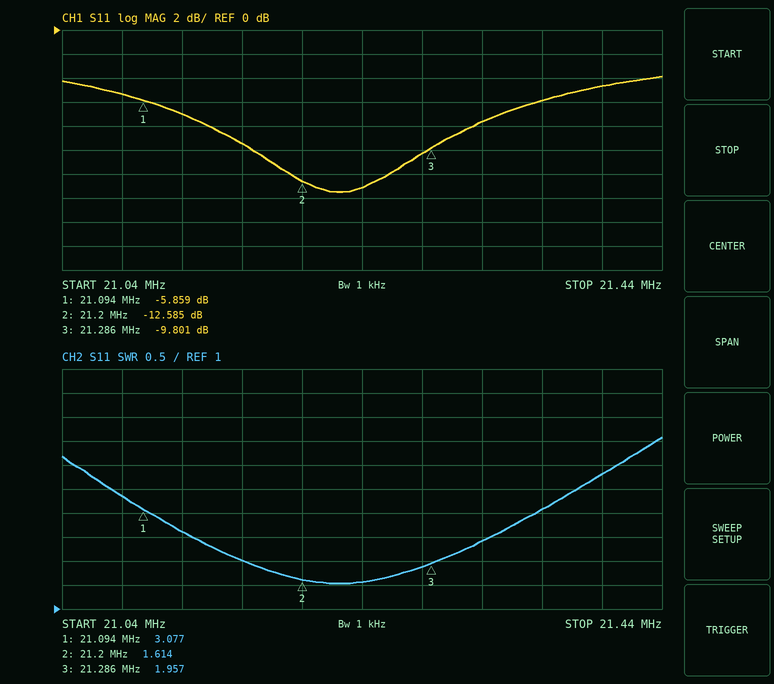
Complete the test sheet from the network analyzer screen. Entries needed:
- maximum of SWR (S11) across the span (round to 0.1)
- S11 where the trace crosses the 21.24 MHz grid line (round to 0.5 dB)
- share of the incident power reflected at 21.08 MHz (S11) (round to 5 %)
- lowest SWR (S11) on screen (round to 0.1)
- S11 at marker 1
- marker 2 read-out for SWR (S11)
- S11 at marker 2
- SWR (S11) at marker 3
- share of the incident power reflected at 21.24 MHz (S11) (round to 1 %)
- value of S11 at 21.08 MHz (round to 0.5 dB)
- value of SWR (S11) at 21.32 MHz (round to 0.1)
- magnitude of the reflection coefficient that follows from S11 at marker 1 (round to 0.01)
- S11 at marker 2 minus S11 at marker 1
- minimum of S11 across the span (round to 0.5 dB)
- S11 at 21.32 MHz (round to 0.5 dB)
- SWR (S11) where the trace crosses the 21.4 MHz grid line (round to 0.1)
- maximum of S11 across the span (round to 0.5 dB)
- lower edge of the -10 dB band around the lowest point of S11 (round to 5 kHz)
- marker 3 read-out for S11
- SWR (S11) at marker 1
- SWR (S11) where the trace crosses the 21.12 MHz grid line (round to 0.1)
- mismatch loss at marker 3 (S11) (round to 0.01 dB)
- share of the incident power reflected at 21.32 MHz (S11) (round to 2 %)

4.6
-13.0 dB
30 %
1.5
-5.859 dB
1.614
-12.585 dB
1.957
5 %
-5.5 dB
2.4
0.51
-6.726 dB
-13.5 dB
-7.5 dB
3.8
-4.0 dB
21.165 MHz
-9.801 dB
3.077
2.6
0.48 dB
18 %
